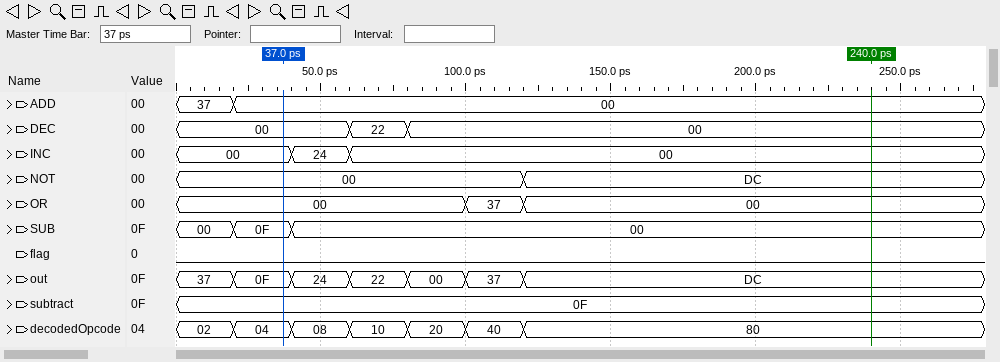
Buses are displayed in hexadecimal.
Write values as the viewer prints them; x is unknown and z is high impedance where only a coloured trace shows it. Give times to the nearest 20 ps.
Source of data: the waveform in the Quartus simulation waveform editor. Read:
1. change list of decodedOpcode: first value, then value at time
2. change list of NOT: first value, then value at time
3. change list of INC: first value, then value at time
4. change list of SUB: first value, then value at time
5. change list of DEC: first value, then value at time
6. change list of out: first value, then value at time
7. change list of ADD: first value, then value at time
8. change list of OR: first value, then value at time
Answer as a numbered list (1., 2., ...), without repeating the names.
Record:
1. 02, 04 at 20 ps, 08 at 40 ps, 10 at 60 ps, 20 at 80 ps, 40 at 100 ps, 80 at 120 ps
2. 00, DC at 120 ps
3. 00, 24 at 40 ps, 00 at 60 ps
4. 00, 0F at 20 ps, 00 at 40 ps
5. 00, 22 at 60 ps, 00 at 80 ps
6. 37, 0F at 20 ps, 24 at 40 ps, 22 at 60 ps, 00 at 80 ps, 37 at 100 ps, DC at 120 ps
7. 37, 00 at 20 ps
8. 00, 37 at 100 ps, 00 at 120 ps
